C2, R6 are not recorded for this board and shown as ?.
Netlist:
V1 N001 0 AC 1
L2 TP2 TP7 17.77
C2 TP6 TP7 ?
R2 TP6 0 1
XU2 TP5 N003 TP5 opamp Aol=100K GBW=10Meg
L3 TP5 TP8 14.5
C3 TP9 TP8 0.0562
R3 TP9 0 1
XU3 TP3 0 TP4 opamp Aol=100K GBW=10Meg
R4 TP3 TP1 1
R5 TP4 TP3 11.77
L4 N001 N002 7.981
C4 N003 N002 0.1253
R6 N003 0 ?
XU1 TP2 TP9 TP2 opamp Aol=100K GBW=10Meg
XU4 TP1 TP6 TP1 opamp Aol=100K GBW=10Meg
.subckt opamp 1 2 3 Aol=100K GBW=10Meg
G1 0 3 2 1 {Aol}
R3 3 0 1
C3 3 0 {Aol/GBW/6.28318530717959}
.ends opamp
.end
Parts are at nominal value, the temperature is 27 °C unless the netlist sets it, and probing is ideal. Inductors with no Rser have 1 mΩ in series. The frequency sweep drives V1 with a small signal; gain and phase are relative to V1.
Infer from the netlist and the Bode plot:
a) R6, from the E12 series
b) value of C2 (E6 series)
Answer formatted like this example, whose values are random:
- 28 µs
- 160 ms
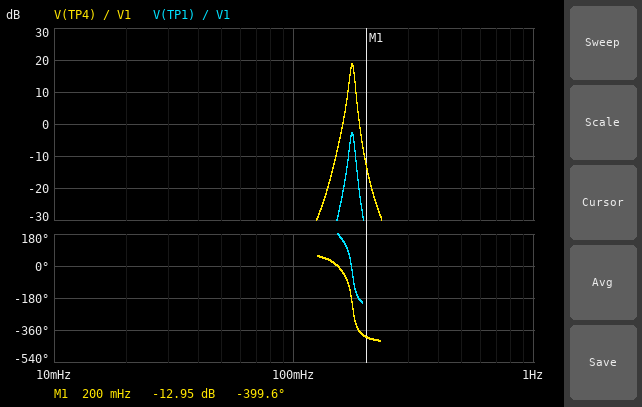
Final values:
- 1.8 Ω
- 47 mF
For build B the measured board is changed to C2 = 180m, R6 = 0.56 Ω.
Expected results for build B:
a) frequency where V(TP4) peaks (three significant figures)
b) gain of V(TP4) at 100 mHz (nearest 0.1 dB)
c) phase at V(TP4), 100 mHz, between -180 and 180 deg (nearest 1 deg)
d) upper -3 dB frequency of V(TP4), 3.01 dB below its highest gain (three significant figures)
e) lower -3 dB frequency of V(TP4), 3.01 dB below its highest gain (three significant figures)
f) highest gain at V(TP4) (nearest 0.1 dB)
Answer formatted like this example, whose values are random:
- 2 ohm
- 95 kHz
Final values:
- 161 mHz
- -35.1 dB
- -74 deg
- 179 mHz
- 156 mHz
- -10.8 dB
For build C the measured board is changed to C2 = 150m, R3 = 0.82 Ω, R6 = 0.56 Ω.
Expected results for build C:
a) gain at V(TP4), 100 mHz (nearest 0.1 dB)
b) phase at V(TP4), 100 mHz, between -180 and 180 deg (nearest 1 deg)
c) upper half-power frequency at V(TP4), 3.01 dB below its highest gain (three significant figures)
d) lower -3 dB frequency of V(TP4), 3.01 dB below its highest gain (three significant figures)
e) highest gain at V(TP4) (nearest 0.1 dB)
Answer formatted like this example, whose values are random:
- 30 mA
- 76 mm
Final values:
- -29.9 dB
- -36 deg
- 179 mHz
- 156 mHz
- -10.8 dB
